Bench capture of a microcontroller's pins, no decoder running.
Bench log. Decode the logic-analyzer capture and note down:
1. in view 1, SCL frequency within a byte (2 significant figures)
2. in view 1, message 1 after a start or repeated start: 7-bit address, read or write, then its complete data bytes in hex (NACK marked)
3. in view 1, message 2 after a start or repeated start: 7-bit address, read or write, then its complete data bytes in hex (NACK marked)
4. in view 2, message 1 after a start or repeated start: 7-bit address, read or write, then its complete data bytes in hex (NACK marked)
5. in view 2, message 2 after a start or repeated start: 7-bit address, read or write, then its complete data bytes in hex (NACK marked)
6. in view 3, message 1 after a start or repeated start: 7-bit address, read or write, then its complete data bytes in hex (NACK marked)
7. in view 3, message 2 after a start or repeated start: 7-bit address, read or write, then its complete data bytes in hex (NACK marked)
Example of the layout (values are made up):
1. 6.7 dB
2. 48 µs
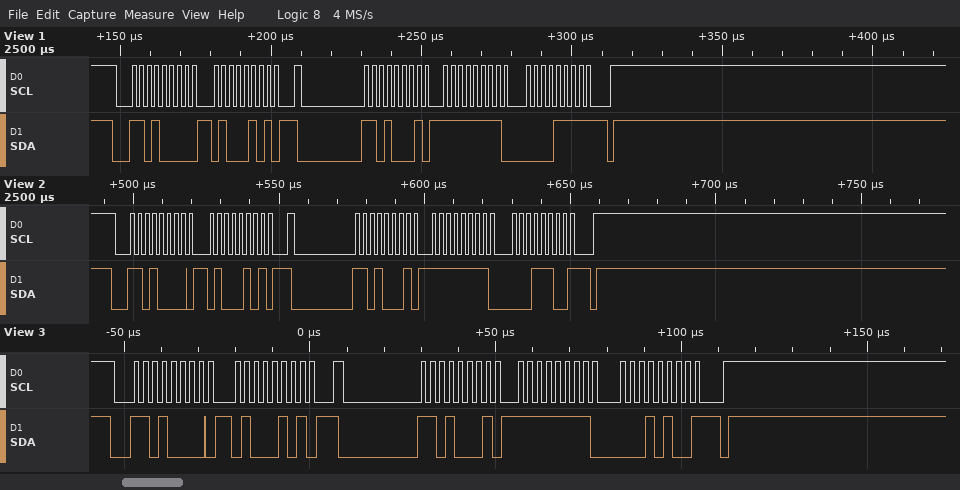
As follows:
1. 400 kHz
2. 0x68 write: 45
3. 0x68 read: FF 0F NACK
4. 0x68 write: 45
5. 0x68 read: FF 1C NACK
6. 0x68 write: 45
7. 0x68 read: FF 14 NACK
